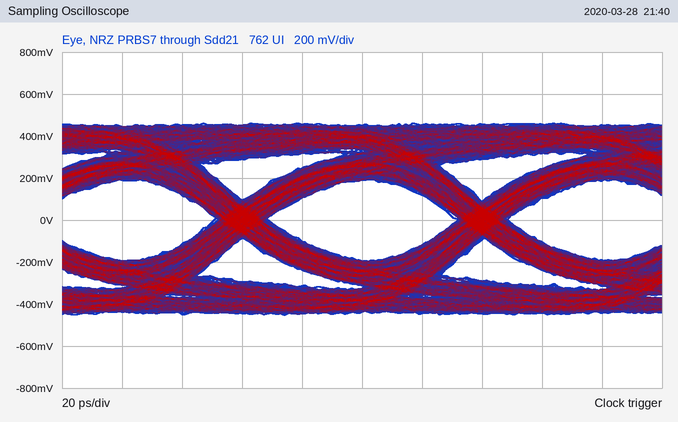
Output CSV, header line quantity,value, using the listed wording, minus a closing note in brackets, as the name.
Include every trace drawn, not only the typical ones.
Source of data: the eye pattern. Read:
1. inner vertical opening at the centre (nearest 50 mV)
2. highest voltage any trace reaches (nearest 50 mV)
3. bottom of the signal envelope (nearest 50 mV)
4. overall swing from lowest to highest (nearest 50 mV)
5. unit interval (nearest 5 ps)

quantity,value
inner vertical opening at the centre,400 mV
highest voltage any trace reaches,450 mV
bottom of the signal envelope,-450 mV
overall swing from lowest to highest,900 mV
unit interval,80 ps
